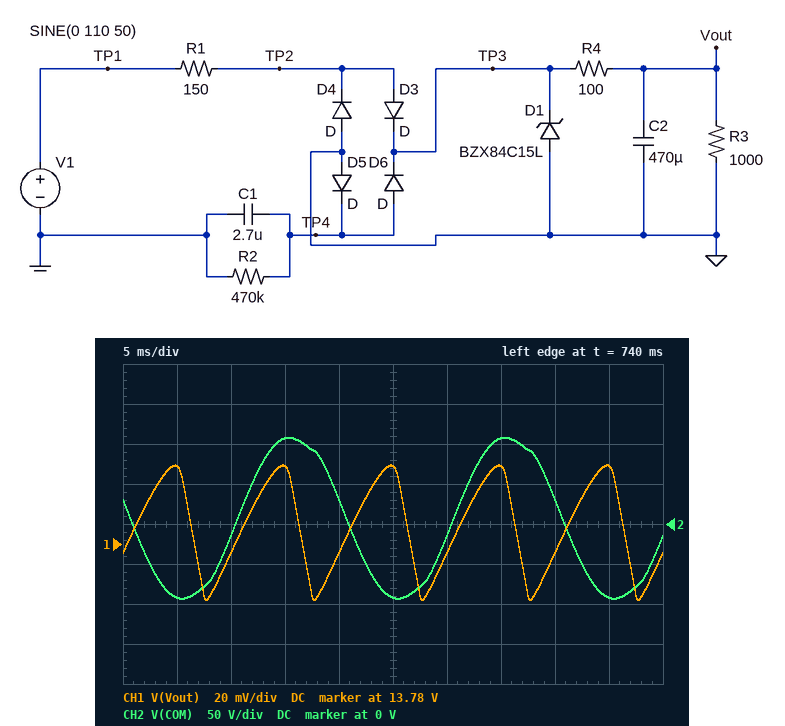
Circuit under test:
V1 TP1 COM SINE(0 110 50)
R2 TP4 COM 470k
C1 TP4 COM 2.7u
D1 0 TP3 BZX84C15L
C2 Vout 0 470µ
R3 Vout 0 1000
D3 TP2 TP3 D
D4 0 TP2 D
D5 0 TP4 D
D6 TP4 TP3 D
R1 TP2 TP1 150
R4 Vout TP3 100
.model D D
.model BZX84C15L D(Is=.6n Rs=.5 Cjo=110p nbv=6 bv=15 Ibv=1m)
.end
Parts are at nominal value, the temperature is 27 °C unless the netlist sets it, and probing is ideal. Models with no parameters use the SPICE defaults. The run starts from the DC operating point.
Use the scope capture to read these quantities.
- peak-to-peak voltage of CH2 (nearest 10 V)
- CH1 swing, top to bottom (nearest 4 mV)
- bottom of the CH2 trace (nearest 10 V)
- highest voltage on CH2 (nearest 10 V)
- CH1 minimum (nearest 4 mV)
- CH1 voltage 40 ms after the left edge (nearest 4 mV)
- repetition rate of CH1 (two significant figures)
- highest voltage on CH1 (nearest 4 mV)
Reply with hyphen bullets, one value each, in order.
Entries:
- 200 V
- 68 mV
- -90 V
- 110 V
- 13.752 V
- 13.776 V
- 100 Hz
- 13.820 V
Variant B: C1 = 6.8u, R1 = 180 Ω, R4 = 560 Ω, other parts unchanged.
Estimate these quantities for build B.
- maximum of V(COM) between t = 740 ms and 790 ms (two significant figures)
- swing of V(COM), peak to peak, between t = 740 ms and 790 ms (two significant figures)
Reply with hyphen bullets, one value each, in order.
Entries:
- 100 V
- 190 V
